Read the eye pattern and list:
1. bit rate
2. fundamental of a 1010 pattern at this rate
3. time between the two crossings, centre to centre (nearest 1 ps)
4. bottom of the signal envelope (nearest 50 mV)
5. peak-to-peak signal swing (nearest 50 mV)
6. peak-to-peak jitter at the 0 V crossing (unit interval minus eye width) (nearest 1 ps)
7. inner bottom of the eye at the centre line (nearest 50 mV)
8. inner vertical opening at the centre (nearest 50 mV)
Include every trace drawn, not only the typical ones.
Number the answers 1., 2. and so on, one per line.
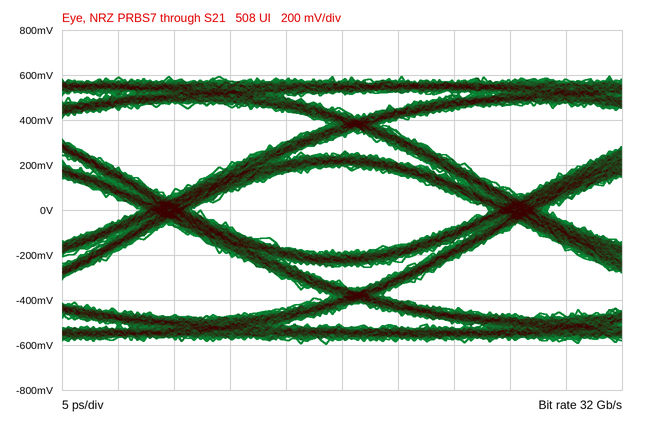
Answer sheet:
1. 32 Gb/s
2. 16 GHz
3. 31 ps
4. -600 mV
5. 1.20 V
6. 5 ps
7. -200 mV
8. 400 mV
